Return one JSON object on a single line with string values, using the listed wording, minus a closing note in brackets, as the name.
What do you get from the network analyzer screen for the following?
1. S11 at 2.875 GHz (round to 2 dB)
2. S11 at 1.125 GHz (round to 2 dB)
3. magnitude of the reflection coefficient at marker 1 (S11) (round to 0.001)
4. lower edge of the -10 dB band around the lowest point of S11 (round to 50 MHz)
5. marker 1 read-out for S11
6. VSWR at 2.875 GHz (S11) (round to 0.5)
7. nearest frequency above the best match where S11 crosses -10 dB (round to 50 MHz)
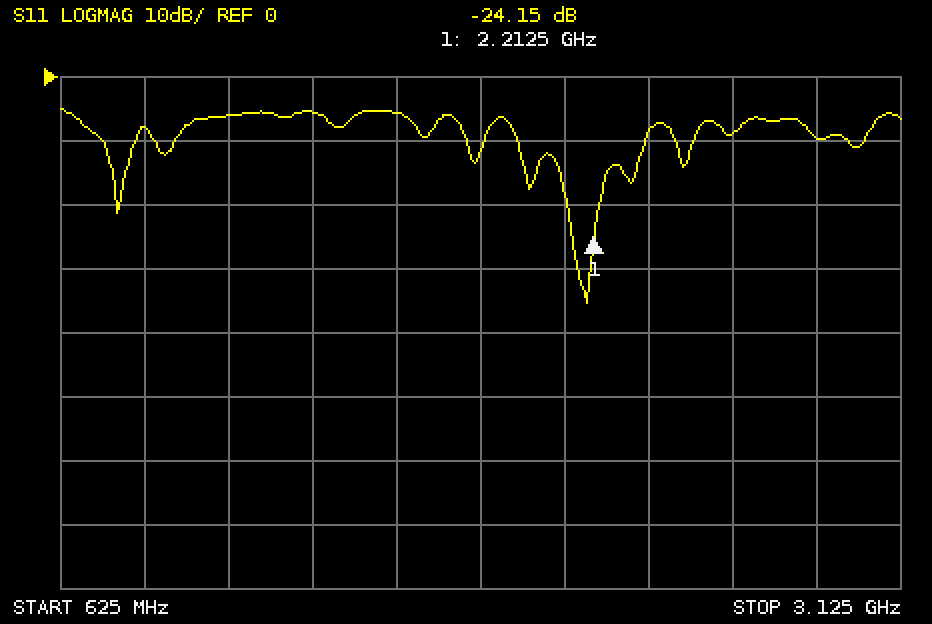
{"S11 at 2.875 GHz": "-10 dB", "S11 at 1.125 GHz": "-6 dB", "magnitude of the reflection coefficient at marker 1 (S11)": "0.062", "lower edge of the -10 dB band around the lowest point of S11": "2.00 GHz", "marker 1 read-out for S11": "-24.15 dB", "VSWR at 2.875 GHz (S11)": "2.0", "nearest frequency above the best match where S11 crosses -10 dB": "2.35 GHz"}
